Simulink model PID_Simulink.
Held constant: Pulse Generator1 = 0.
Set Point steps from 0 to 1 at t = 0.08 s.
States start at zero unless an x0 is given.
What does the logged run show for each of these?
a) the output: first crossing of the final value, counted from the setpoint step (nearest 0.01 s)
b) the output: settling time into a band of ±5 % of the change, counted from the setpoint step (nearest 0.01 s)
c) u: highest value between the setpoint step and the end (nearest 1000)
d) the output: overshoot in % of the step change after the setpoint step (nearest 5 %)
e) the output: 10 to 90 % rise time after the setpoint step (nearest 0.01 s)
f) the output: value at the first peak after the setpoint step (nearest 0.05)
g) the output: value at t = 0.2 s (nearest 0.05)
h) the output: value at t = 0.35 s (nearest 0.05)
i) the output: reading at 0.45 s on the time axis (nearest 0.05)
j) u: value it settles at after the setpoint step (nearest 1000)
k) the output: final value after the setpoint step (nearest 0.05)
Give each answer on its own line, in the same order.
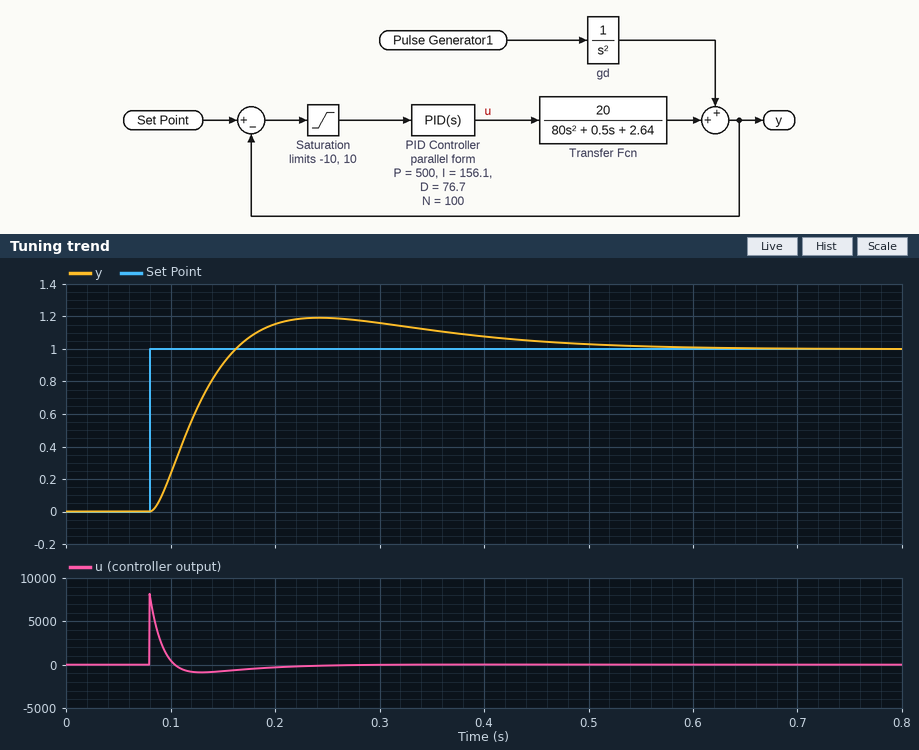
0.08 s
0.37 s
8000
20 %
0.06 s
1.20
1.15
1.10
1.05
0
1.00
